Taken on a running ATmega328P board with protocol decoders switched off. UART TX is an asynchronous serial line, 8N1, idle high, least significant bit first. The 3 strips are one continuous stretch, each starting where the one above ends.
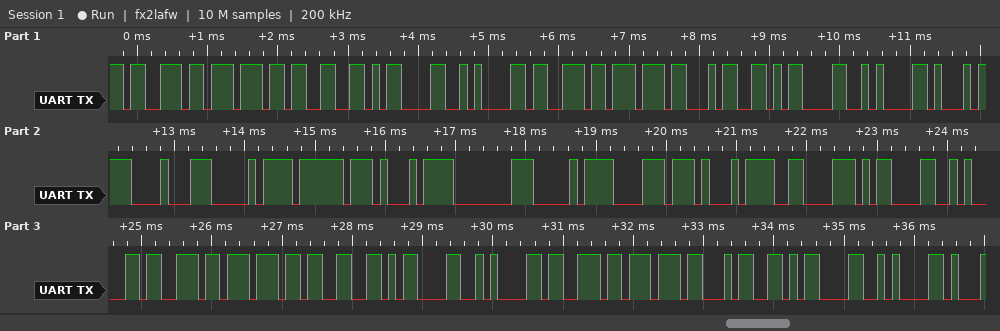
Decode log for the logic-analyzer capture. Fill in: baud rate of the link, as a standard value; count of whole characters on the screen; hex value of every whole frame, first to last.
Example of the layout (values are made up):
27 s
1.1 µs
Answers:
9600 baud
32
0x73 0x77 0x33 0x0D 0x0A 0x73 0x77 0x34 0x0D 0x0A 0xD1 0x88 0xD0 0xBF 0xD1 0x80 0xD0 0xB8 0xD1 0x86 0x0D 0x0A 0x73 0x77 0x33 0x0D 0x0A 0x73 0x77 0x34 0x0D 0x0A
